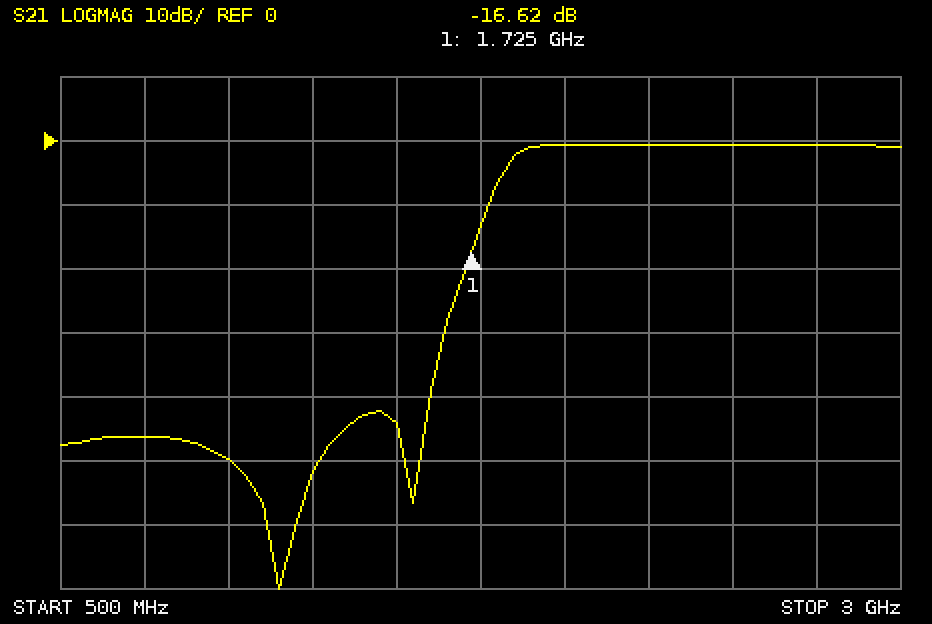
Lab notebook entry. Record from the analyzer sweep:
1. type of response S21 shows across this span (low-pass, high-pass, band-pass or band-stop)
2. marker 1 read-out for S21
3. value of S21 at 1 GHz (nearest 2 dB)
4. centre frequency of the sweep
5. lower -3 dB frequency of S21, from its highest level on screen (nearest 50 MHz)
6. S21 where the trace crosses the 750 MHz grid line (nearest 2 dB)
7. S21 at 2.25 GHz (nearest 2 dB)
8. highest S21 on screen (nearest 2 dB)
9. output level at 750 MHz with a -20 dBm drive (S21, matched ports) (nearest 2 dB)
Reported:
high-pass
-16.62 dB
-50 dB
1.75 GHz
1.85 GHz
-46 dB
0 dB
0 dB
-66 dBm
